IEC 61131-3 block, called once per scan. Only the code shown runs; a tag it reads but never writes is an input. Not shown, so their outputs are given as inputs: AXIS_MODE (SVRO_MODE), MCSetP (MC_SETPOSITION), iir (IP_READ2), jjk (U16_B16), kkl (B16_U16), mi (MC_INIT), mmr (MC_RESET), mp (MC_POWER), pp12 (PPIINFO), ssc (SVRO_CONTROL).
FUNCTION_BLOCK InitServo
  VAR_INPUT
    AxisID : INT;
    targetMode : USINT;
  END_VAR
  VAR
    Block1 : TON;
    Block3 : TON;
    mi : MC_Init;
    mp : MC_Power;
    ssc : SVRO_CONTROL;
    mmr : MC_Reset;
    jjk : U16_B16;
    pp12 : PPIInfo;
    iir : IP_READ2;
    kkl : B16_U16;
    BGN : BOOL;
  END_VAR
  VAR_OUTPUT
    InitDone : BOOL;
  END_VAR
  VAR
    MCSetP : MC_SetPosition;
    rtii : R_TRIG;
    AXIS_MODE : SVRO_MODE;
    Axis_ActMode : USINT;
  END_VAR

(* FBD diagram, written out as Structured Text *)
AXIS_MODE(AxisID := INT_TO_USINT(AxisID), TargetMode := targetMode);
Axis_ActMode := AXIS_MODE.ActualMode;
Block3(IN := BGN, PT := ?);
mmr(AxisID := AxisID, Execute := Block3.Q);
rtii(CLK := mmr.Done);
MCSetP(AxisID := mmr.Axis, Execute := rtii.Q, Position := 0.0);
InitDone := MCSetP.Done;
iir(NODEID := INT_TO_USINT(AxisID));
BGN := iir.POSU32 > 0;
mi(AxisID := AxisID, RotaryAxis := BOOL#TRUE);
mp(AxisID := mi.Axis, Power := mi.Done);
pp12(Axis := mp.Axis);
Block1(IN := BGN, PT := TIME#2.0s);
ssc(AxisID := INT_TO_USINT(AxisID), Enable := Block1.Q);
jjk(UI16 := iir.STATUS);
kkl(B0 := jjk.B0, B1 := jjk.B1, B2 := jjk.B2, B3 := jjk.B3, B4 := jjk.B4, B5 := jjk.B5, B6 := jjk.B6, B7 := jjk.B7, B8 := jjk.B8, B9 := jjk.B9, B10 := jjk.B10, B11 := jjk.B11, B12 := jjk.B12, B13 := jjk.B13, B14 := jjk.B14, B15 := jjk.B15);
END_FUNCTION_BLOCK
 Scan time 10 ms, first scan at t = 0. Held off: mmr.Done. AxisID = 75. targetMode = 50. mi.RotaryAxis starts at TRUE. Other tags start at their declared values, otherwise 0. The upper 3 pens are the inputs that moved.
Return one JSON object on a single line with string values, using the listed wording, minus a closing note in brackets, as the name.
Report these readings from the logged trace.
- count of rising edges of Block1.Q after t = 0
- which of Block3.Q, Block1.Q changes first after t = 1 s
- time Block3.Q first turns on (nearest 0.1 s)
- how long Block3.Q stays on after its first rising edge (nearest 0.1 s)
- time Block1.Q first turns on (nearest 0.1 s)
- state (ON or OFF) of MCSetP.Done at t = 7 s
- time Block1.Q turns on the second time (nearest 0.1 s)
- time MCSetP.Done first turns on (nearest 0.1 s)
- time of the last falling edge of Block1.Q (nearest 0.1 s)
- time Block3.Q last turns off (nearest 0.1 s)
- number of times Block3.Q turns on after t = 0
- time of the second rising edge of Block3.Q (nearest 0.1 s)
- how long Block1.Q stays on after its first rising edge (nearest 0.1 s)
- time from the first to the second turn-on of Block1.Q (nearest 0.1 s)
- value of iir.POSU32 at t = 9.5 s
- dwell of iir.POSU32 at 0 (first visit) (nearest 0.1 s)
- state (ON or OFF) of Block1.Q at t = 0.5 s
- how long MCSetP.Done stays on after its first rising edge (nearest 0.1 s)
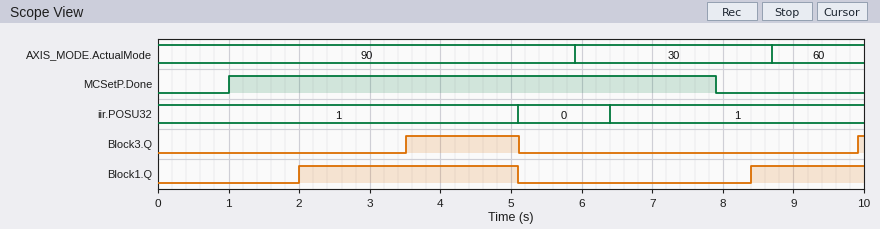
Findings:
{"count of rising edges of Block1.Q after t = 0": "2", "which of Block3.Q, Block1.Q changes first after t = 1 s": "Block1.Q", "time Block3.Q first turns on": "3.5 s", "how long Block3.Q stays on after its first rising edge": "1.6 s", "time Block1.Q first turns on": "2.0 s", "state (ON or OFF) of MCSetP.Done at t = 7 s": "ON", "time Block1.Q turns on the second time": "8.4 s", "time MCSetP.Done first turns on": "1.0 s", "time of the last falling edge of Block1.Q": "5.1 s", "time Block3.Q last turns off": "5.1 s", "number of times Block3.Q turns on after t = 0": "2", "time of the second rising edge of Block3.Q": "9.9 s", "how long Block1.Q stays on after its first rising edge": "3.1 s", "time from the first to the second turn-on of Block1.Q": "6.4 s", "value of iir.POSU32 at t = 9.5 s": "1", "dwell of iir.POSU32 at 0 (first visit)": "1.3 s", "state (ON or OFF) of Block1.Q at t = 0.5 s": "OFF", "how long MCSetP.Done stays on after its first rising edge": "6.9 s"}
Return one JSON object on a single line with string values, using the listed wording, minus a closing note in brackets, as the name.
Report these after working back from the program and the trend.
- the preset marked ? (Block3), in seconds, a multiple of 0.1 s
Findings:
{"the preset marked ? (Block3), in seconds, a multiple of 0.1 s": "3.5 s"}
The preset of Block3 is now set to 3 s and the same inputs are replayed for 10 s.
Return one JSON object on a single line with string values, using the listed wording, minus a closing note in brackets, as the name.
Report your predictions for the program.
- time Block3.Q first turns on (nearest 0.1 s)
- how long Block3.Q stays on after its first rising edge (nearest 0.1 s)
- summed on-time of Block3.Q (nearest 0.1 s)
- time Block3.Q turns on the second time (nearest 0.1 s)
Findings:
{"time Block3.Q first turns on": "3.0 s", "how long Block3.Q stays on after its first rising edge": "2.1 s", "summed on-time of Block3.Q": "2.7 s", "time Block3.Q turns on the second time": "9.4 s"}
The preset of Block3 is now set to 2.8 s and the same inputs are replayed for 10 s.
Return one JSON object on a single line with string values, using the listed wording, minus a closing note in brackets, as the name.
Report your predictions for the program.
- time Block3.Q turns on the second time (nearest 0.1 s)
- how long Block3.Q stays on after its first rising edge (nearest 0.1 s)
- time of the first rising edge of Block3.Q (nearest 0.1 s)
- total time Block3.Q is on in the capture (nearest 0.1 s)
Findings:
{"time Block3.Q turns on the second time": "9.2 s", "how long Block3.Q stays on after its first rising edge": "2.3 s", "time of the first rising edge of Block3.Q": "2.8 s", "total time Block3.Q is on in the capture": "3.1 s"}
